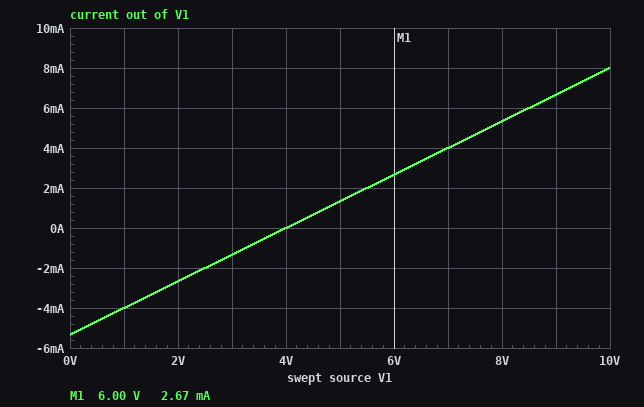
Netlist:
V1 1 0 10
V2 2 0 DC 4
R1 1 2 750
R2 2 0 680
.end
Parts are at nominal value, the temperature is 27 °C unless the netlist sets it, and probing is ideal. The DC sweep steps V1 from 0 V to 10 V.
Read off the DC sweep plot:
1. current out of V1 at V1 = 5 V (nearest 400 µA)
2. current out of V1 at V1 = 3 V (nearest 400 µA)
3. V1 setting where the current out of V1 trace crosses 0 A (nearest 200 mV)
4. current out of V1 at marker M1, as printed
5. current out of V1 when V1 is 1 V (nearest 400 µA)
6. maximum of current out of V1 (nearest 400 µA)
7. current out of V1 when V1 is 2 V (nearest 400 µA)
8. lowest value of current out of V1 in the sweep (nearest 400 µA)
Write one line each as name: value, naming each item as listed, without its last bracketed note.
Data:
current out of V1 at V1 = 5 V: 1.2 mA
current out of V1 at V1 = 3 V: -1.2 mA
V1 setting where the current out of V1 trace crosses 0 A: 4.0 V
current out of V1 at marker M1, as printed: 2.67 mA
current out of V1 when V1 is 1 V: -4.0 mA
maximum of current out of V1: 8.0 mA
current out of V1 when V1 is 2 V: -2.8 mA
lowest value of current out of V1 in the sweep: -5.2 mA
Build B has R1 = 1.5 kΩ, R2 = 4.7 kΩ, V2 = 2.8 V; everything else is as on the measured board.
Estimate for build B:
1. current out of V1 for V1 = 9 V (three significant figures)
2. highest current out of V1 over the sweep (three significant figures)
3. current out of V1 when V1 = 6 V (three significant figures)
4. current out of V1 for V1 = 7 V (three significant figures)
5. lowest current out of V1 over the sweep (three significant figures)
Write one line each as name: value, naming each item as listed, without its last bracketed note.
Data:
current out of V1 for V1 = 9 V: 4.13 mA
highest current out of V1 over the sweep: 4.80 mA
current out of V1 when V1 = 6 V: 2.13 mA
current out of V1 for V1 = 7 V: 2.80 mA
lowest current out of V1 over the sweep: -1.87 mA
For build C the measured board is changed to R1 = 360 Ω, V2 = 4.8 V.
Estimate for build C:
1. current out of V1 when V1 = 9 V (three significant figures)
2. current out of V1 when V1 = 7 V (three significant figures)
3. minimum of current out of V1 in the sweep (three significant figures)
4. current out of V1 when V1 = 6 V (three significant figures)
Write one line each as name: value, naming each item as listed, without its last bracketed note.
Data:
current out of V1 when V1 = 9 V: 11.7 mA
current out of V1 when V1 = 7 V: 6.11 mA
minimum of current out of V1 in the sweep: -13.3 mA
current out of V1 when V1 = 6 V: 3.33 mA
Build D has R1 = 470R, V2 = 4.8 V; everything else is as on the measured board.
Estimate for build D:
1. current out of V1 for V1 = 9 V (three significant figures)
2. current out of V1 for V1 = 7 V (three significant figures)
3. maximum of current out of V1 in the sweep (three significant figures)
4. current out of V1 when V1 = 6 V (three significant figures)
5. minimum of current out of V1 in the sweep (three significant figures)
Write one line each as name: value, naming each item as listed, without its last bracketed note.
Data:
current out of V1 for V1 = 9 V: 8.94 mA
current out of V1 for V1 = 7 V: 4.68 mA
maximum of current out of V1 in the sweep: 11.1 mA
current out of V1 when V1 = 6 V: 2.55 mA
minimum of current out of V1 in the sweep: -10.2 mA
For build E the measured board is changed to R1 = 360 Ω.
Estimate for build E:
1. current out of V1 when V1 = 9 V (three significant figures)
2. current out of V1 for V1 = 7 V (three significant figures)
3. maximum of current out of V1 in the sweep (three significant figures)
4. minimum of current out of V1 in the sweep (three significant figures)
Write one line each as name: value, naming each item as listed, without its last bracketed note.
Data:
current out of V1 when V1 = 9 V: 13.9 mA
current out of V1 for V1 = 7 V: 8.33 mA
maximum of current out of V1 in the sweep: 16.7 mA
minimum of current out of V1 in the sweep: -11.1 mA
